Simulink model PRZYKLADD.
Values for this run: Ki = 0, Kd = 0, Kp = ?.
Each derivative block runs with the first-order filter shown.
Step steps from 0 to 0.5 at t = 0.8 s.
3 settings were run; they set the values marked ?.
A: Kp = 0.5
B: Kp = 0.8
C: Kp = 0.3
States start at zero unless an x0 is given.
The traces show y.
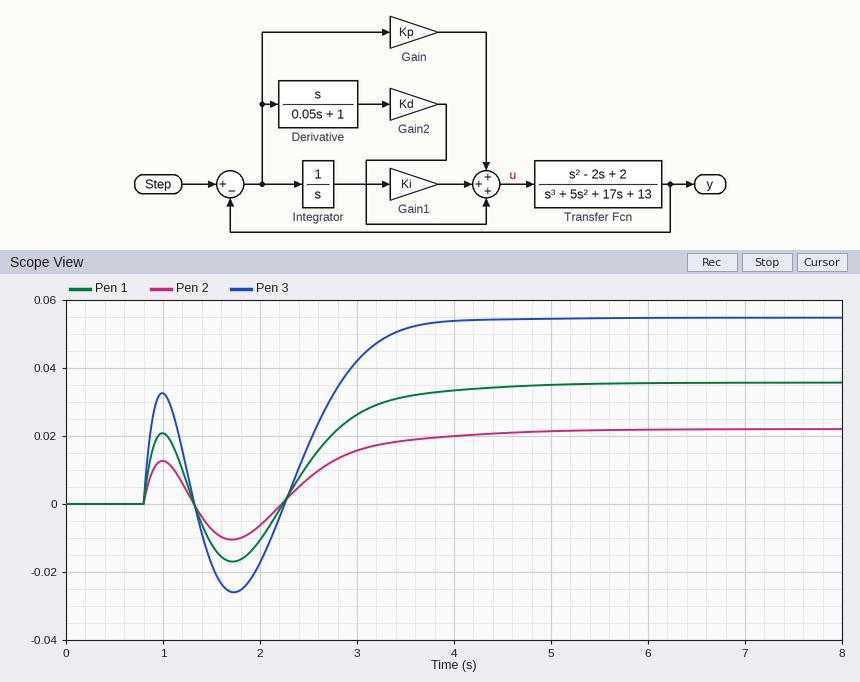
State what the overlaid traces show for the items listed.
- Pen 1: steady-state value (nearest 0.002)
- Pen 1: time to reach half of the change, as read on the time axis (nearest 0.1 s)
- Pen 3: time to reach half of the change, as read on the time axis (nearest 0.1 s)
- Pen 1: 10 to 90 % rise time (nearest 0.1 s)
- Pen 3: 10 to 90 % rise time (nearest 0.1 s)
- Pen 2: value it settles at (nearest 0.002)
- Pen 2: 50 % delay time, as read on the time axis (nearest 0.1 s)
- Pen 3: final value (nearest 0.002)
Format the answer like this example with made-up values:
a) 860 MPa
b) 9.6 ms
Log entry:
a) 0.036
b) 0.9 s
c) 0.9 s
d) 2.8 s
e) 2.5 s
f) 0.022
g) 0.9 s
h) 0.054
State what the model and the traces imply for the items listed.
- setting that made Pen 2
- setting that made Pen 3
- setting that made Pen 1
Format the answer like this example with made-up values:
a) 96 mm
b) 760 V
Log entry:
a) C
b) B
c) A
